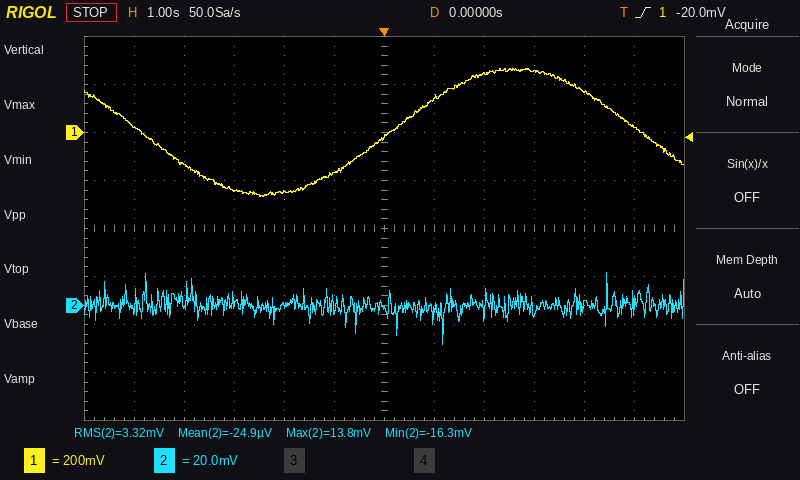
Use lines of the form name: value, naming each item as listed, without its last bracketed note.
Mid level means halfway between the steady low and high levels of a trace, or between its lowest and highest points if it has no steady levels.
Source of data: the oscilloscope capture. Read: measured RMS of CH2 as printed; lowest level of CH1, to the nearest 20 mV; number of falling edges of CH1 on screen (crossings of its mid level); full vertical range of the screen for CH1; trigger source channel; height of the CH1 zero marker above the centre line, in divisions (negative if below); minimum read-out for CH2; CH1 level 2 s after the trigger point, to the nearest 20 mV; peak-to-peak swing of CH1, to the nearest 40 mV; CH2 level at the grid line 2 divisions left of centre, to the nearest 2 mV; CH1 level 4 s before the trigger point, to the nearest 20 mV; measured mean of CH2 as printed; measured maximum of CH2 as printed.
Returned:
measured RMS of CH2 as printed: 3.32 mV
lowest level of CH1, to the nearest 20 mV: -260 mV
number of falling edges of CH1 on screen: 2
full vertical range of the screen for CH1: 1.6 V
trigger source channel: CH1
height of the CH1 zero marker above the centre line, in divisions: +2.0 div
minimum read-out for CH2: -16.3 mV
CH1 level 2 s after the trigger point, to the nearest 20 mV: 240 mV
peak-to-peak swing of CH1, to the nearest 40 mV: 520 mV
CH2 level at the grid line 2 divisions left of centre, to the nearest 2 mV: 0 mV
CH1 level 4 s before the trigger point, to the nearest 20 mV: -140 mV
measured mean of CH2 as printed: -24.9 µV
measured maximum of CH2 as printed: 13.8 mV
